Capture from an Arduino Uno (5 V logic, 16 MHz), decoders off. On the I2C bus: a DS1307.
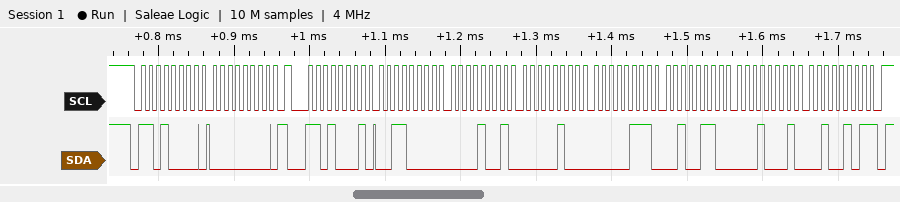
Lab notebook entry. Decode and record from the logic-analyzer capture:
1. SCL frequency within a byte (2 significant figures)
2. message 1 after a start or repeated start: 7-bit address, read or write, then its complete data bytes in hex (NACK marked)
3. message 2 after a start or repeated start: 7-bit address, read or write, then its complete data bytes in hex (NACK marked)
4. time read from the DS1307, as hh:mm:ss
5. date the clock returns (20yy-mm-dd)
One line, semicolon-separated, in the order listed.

100 kHz; 0x68 write: 00; 0x68 read: 30 09 04 07 26 11 25 NACK; 04:09:30; 2025-11-26
